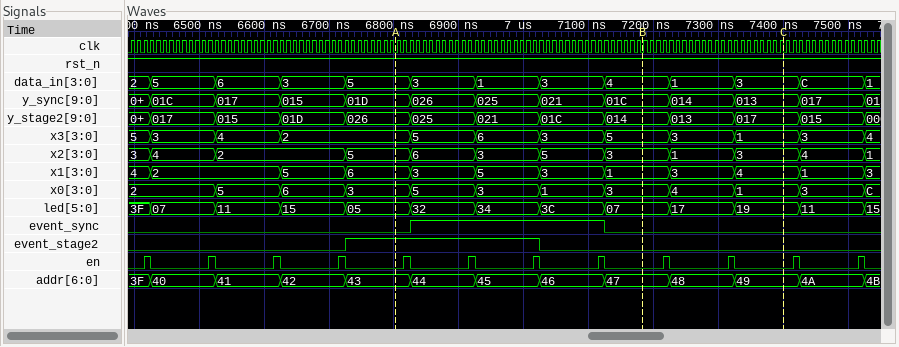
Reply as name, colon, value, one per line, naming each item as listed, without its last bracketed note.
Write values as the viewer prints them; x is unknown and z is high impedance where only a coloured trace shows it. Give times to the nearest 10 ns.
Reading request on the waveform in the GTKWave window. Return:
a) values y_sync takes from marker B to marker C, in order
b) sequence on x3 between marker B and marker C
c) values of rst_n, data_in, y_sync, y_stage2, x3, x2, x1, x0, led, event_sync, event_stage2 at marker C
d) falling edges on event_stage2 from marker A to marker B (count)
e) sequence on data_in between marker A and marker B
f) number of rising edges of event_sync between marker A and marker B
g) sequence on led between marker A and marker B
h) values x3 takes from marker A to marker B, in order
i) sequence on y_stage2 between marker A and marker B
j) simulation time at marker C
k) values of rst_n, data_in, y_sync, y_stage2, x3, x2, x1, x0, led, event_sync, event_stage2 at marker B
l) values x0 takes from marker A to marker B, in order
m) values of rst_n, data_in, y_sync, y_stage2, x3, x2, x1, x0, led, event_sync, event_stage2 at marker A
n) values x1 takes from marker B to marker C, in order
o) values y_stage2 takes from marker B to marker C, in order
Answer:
values y_sync takes from marker B to marker C, in order: 01C, 014, 013
sequence on x3 between marker B and marker C: 5, 3, 1
values of rst_n, data_in, y_sync, y_stage2, x3, x2, x1, x0, led, event_sync, event_stage2 at marker C: rst_n=1, data_in=3, y_sync=013, y_stage2=017, x3=1, x2=3, x1=4, x0=1, led=19, event_sync=0, event_stage2=0
falling edges on event_stage2 from marker A to marker B: 1
sequence on data_in between marker A and marker B: 5, 3, 1, 3, 4
number of rising edges of event_sync between marker A and marker B: 1
sequence on led between marker A and marker B: 05, 32, 34, 3C, 07
values x3 takes from marker A to marker B, in order: 2, 5, 6, 3, 5
sequence on y_stage2 between marker A and marker B: 026, 025, 021, 01C, 014
simulation time at marker C: 7400 ns
values of rst_n, data_in, y_sync, y_stage2, x3, x2, x1, x0, led, event_sync, event_stage2 at marker B: rst_n=1, data_in=4, y_sync=01C, y_stage2=014, x3=5, x2=3, x1=1, x0=3, led=07, event_sync=0, event_stage2=0
values x0 takes from marker A to marker B, in order: 3, 5, 3, 1, 3
values of rst_n, data_in, y_sync, y_stage2, x3, x2, x1, x0, led, event_sync, event_stage2 at marker A: rst_n=1, data_in=5, y_sync=01D, y_stage2=026, x3=2, x2=5, x1=6, x0=3, led=05, event_sync=0, event_stage2=1
values x1 takes from marker B to marker C, in order: 1, 3, 4
values y_stage2 takes from marker B to marker C, in order: 014, 013, 017
